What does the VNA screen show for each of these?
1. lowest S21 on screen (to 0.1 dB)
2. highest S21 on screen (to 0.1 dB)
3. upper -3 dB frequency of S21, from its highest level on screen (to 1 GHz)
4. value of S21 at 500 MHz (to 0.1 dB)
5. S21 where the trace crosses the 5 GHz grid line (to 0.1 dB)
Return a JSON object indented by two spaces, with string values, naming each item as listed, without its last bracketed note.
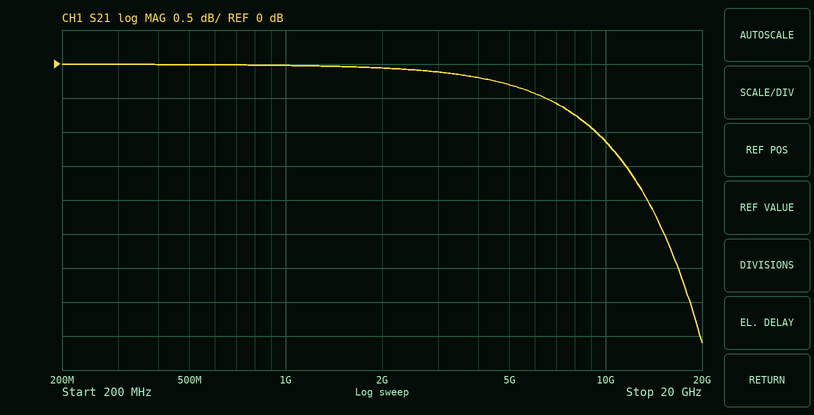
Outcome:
{
  "lowest S21 on screen": "-4.1 dB",
  "highest S21 on screen": "0.0 dB",
  "upper -3 dB frequency of S21, from its highest level on screen": "17 GHz",
  "value of S21 at 500 MHz": "0.0 dB",
  "S21 where the trace crosses the 5 GHz grid line": "-0.3 dB"
}
